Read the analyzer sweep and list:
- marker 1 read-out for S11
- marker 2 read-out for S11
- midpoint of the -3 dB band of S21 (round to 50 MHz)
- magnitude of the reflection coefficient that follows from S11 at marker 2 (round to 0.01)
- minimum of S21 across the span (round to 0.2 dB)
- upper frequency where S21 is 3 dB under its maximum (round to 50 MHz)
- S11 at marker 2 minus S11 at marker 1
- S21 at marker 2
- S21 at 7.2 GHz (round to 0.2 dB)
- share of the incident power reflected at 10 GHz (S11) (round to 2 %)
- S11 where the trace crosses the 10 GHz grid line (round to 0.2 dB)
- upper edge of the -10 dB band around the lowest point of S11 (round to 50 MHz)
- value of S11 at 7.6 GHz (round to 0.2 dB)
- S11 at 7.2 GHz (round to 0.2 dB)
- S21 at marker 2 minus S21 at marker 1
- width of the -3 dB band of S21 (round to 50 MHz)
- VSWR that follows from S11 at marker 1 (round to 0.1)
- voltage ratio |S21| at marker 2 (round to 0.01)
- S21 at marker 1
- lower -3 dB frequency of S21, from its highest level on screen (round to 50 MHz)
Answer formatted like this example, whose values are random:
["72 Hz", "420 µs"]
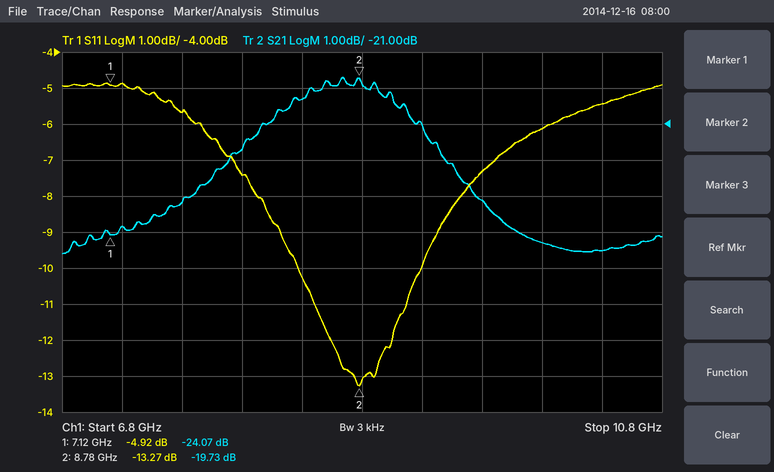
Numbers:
["-4.92 dB", "-13.27 dB", "8.60 GHz", "0.22", "-24.6 dB", "9.50 GHz", "-8.35 dB", "-19.73 dB", "-23.8 dB", "24 %", "-6.2 dB", "9.20 GHz", "-5.6 dB", "-4.8 dB", "4.34 dB", "1.80 GHz", "3.6", "0.10", "-24.07 dB", "7.70 GHz"]
